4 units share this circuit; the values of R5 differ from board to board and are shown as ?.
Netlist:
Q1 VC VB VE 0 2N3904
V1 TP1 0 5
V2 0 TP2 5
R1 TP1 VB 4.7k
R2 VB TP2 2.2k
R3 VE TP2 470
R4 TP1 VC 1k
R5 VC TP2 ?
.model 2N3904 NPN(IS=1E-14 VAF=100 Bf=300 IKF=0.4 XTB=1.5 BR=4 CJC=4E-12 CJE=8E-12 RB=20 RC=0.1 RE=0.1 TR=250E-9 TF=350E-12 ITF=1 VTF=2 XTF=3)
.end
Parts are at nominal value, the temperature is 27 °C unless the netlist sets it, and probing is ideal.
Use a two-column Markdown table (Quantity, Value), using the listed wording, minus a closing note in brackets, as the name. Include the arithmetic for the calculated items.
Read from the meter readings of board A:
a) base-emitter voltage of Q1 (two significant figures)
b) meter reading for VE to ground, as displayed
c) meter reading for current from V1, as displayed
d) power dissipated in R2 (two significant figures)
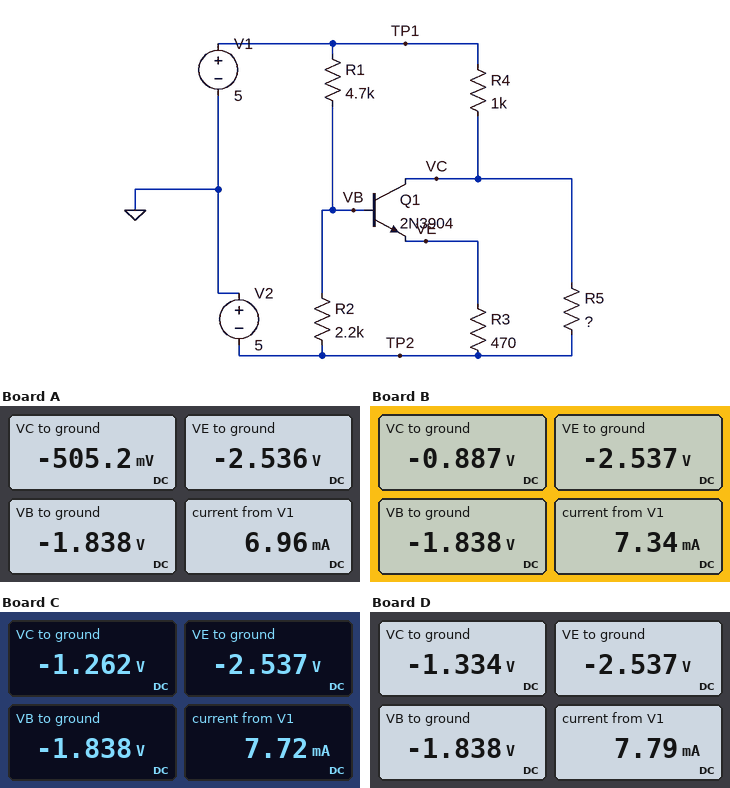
| Quantity | Value |
|---|---|
| base-emitter voltage of Q1 | -1.838 V - (-2.536 V) = 700 mV |
| meter reading for VE to ground, as displayed | -2.536 V |
| meter reading for current from V1, as displayed | 6.96 mA |
| power dissipated in R2 | (-1.838 V - (-5 V))^2 / 2.2 kΩ = 4.5 mW |
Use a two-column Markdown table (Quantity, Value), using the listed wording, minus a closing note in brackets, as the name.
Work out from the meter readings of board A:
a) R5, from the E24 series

| Quantity | Value |
|---|---|
| R5, from the E24 series | 16 kΩ |
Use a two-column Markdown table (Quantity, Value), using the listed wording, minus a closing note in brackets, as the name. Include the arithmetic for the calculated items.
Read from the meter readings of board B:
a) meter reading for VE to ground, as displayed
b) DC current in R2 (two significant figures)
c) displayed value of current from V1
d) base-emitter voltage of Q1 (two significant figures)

| Quantity | Value |
|---|---|
| meter reading for VE to ground, as displayed | -2.537 V |
| DC current in R2 | (-1.838 V - (-5 V)) / 2.2 kΩ = 1.4 mA |
| displayed value of current from V1 | 7.34 mA |
| base-emitter voltage of Q1 | -1.838 V - (-2.537 V) = 700 mV |
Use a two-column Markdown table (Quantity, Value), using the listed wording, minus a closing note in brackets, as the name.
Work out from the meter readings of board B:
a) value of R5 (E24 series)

| Quantity | Value |
|---|---|
| value of R5 | 6.2 kΩ |
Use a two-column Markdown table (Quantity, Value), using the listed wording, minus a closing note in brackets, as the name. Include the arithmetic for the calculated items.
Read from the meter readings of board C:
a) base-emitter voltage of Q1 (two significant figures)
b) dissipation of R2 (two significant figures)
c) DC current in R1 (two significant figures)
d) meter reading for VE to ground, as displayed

| Quantity | Value |
|---|---|
| base-emitter voltage of Q1 | -1.838 V - (-2.537 V) = 700 mV |
| dissipation of R2 | (-1.838 V - (-5 V))^2 / 2.2 kΩ = 4.5 mW |
| DC current in R1 | (5 V - (-1.838 V)) / 4.7 kΩ = 1.5 mA |
| meter reading for VE to ground, as displayed | -2.537 V |
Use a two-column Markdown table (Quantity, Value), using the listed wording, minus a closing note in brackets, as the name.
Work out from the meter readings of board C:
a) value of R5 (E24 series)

| Quantity | Value |
|---|---|
| value of R5 | 3.6 kΩ |
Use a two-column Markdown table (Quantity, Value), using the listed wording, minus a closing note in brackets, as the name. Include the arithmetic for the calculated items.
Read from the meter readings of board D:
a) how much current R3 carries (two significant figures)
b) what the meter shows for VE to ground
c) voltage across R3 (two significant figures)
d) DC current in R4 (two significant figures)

| Quantity | Value |
|---|---|
| how much current R3 carries | (-2.537 V - (-5 V)) / 470 Ω = 5.2 mA |
| what the meter shows for VE to ground | -2.537 V |
| voltage across R3 | -2.537 V - (-5 V) = 2.5 V |
| DC current in R4 | (5 V - (-1.334 V)) / 1 kΩ = 6.3 mA |
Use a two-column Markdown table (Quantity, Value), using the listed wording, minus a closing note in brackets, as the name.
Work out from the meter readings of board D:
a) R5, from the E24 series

| Quantity | Value |
|---|---|
| R5, from the E24 series | 3.3 kΩ |
